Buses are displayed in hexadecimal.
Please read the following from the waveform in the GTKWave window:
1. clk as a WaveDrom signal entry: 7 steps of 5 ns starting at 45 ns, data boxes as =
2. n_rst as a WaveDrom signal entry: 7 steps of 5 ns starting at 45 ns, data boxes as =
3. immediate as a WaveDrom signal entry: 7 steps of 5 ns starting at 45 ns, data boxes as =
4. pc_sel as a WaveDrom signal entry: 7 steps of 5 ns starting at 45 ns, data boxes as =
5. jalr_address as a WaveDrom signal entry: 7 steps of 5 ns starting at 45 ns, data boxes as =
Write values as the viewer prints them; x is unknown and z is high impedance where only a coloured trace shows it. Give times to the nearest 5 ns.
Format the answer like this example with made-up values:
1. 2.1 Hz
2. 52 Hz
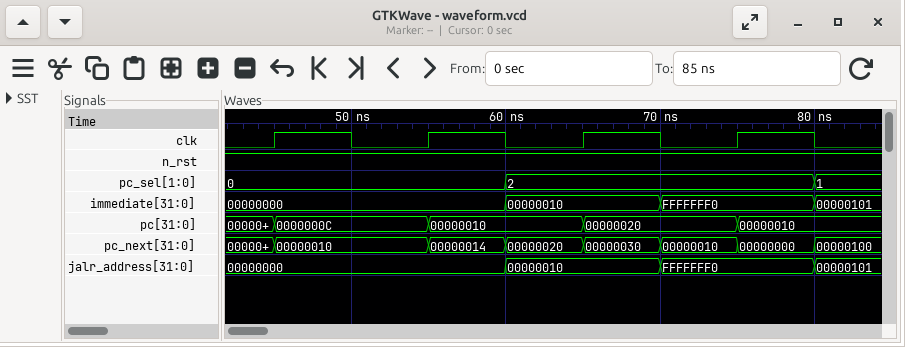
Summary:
1. {name: 'clk', wave: '1010101'}
2. {name: 'n_rst', wave: '1......'}
3. {name: 'immediate', wave: '=..=.=.', data: '00000000 00000010 FFFFFFF0'}
4. {name: 'pc_sel', wave: '=..=...', data: '0 2'}
5. {name: 'jalr_address', wave: '=..=.=.', data: '00000000 00000010 FFFFFFF0'}
